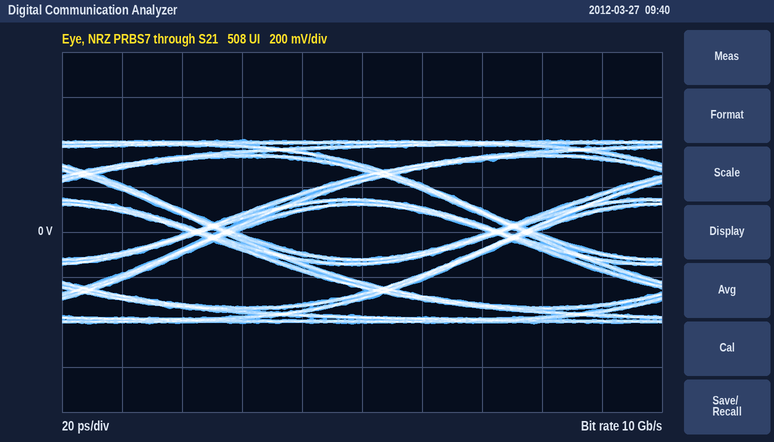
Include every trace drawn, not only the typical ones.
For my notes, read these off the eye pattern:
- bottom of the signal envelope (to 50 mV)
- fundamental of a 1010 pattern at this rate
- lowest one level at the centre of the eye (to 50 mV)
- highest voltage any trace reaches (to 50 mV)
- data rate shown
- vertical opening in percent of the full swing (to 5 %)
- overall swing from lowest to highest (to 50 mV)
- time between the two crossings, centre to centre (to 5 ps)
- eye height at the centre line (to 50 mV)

-400 mV
5 GHz
100 mV
400 mV
10 Gb/s
30 %
800 mV
100 ps
250 mV
